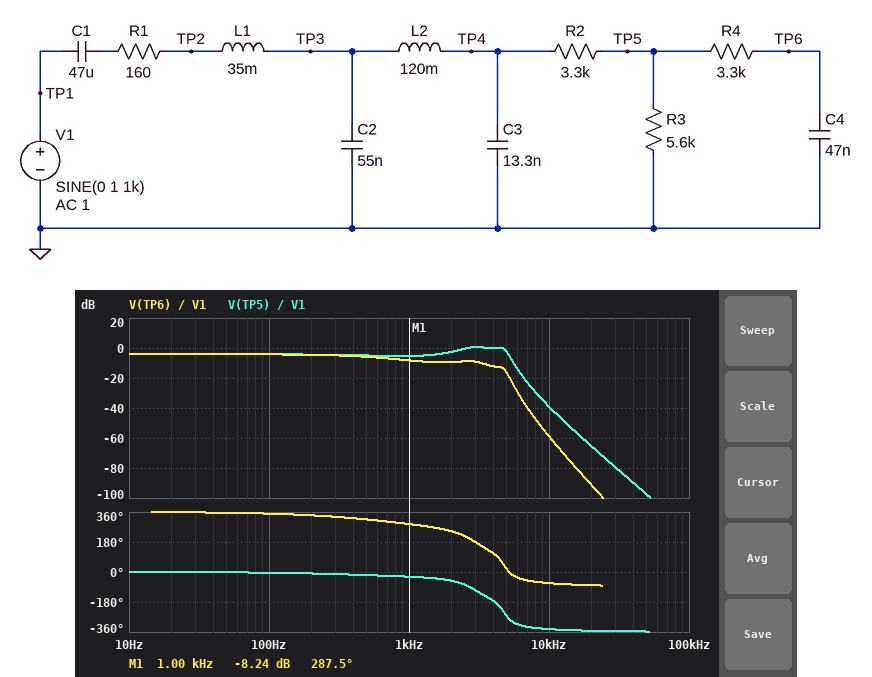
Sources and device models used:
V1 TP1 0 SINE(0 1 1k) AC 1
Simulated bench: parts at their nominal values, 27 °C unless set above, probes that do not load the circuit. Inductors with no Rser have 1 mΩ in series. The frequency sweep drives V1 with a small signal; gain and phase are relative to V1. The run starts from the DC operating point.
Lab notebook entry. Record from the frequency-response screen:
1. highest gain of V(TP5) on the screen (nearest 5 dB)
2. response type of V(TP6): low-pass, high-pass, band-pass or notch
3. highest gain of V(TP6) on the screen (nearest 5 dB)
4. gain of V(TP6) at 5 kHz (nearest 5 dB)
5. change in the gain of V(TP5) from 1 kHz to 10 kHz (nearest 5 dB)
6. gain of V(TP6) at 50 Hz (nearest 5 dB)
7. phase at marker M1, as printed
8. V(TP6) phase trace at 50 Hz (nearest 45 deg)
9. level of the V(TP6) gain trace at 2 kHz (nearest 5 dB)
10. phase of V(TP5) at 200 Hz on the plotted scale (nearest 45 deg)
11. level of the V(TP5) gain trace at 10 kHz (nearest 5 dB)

0 dB
low-pass
-5 dB
-15 dB
-35 dB
-5 dB
287.5 deg
360 deg
-10 dB
0 deg
-40 dB
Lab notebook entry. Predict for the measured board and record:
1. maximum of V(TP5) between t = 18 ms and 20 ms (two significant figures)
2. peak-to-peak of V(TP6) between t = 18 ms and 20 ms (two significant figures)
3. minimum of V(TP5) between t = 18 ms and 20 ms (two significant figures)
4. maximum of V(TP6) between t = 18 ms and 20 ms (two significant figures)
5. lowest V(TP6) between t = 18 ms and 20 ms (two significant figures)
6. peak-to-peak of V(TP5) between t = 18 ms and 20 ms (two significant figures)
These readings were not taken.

540 mV
770 mV
-540 mV
390 mV
-390 mV
1.1 V
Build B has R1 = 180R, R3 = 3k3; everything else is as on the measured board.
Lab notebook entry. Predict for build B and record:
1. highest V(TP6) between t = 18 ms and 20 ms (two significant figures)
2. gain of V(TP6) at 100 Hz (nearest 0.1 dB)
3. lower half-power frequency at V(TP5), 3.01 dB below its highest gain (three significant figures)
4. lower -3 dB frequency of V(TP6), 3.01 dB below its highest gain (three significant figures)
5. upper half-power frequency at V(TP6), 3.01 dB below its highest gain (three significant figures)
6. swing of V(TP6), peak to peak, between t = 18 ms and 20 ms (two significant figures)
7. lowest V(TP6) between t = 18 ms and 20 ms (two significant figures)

320 mV
-6.3 dB
2.00 kHz
498 mHz
830 Hz
640 mV
-320 mV
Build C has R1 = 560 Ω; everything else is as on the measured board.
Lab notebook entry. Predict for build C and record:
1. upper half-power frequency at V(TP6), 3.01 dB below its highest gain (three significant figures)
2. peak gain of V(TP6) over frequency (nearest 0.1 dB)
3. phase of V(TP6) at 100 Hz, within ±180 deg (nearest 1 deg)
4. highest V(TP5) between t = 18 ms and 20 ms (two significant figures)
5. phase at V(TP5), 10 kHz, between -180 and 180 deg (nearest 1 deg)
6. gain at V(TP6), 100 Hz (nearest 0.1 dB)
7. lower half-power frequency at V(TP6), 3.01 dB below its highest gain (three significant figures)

687 Hz
-4.6 dB
-11 deg
480 mV
29 deg
-4.7 dB
357 mHz
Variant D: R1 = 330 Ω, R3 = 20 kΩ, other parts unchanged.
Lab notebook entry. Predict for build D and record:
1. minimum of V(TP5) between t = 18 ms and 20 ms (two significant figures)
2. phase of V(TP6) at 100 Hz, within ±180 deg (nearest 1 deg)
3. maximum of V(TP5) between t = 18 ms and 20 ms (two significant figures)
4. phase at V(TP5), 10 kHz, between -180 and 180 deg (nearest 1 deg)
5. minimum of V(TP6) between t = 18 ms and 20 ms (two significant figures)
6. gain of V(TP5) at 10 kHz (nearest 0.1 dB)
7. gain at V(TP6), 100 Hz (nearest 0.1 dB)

-660 mV
-12 deg
660 mV
20 deg
-470 mV
-37.5 dB
-1.6 dB
